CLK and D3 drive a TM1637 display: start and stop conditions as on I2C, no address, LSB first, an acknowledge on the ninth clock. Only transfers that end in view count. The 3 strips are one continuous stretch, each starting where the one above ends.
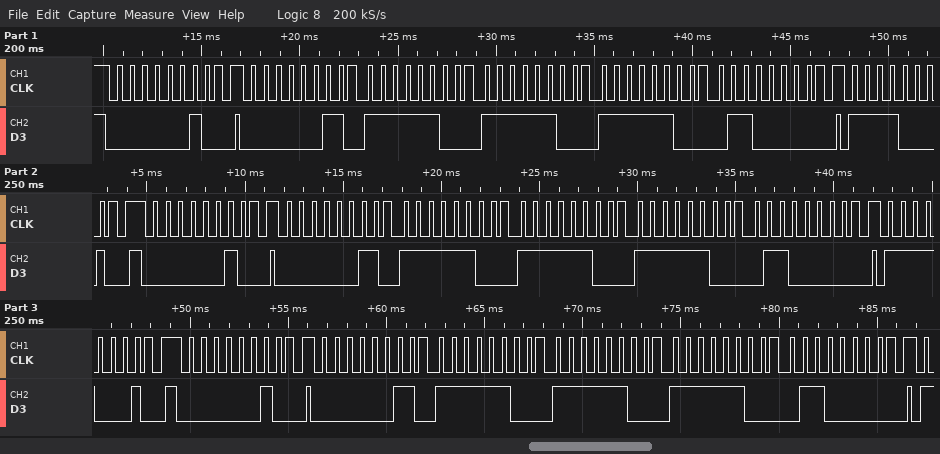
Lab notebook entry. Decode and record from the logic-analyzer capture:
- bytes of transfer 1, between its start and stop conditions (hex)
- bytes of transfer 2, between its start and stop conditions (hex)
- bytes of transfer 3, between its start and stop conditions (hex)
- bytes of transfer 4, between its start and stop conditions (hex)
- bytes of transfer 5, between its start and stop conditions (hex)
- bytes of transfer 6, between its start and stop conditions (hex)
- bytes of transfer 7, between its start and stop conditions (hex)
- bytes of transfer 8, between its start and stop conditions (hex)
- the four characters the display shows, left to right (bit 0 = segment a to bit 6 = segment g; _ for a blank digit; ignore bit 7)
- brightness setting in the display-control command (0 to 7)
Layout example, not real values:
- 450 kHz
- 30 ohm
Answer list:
- 40
- C0 3F 3F 3F 06
- 8F
- 40
- C0 3F 3F 3F 06
- 8F
- 40
- C0 3F 3F 3F 06
- 0001
- 7
